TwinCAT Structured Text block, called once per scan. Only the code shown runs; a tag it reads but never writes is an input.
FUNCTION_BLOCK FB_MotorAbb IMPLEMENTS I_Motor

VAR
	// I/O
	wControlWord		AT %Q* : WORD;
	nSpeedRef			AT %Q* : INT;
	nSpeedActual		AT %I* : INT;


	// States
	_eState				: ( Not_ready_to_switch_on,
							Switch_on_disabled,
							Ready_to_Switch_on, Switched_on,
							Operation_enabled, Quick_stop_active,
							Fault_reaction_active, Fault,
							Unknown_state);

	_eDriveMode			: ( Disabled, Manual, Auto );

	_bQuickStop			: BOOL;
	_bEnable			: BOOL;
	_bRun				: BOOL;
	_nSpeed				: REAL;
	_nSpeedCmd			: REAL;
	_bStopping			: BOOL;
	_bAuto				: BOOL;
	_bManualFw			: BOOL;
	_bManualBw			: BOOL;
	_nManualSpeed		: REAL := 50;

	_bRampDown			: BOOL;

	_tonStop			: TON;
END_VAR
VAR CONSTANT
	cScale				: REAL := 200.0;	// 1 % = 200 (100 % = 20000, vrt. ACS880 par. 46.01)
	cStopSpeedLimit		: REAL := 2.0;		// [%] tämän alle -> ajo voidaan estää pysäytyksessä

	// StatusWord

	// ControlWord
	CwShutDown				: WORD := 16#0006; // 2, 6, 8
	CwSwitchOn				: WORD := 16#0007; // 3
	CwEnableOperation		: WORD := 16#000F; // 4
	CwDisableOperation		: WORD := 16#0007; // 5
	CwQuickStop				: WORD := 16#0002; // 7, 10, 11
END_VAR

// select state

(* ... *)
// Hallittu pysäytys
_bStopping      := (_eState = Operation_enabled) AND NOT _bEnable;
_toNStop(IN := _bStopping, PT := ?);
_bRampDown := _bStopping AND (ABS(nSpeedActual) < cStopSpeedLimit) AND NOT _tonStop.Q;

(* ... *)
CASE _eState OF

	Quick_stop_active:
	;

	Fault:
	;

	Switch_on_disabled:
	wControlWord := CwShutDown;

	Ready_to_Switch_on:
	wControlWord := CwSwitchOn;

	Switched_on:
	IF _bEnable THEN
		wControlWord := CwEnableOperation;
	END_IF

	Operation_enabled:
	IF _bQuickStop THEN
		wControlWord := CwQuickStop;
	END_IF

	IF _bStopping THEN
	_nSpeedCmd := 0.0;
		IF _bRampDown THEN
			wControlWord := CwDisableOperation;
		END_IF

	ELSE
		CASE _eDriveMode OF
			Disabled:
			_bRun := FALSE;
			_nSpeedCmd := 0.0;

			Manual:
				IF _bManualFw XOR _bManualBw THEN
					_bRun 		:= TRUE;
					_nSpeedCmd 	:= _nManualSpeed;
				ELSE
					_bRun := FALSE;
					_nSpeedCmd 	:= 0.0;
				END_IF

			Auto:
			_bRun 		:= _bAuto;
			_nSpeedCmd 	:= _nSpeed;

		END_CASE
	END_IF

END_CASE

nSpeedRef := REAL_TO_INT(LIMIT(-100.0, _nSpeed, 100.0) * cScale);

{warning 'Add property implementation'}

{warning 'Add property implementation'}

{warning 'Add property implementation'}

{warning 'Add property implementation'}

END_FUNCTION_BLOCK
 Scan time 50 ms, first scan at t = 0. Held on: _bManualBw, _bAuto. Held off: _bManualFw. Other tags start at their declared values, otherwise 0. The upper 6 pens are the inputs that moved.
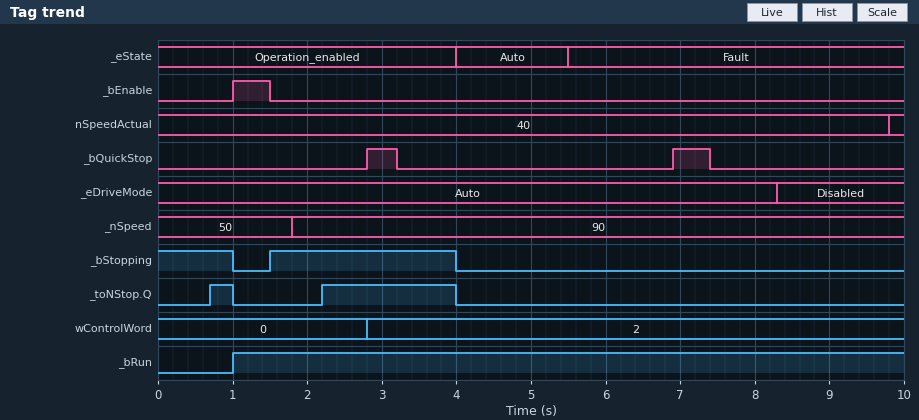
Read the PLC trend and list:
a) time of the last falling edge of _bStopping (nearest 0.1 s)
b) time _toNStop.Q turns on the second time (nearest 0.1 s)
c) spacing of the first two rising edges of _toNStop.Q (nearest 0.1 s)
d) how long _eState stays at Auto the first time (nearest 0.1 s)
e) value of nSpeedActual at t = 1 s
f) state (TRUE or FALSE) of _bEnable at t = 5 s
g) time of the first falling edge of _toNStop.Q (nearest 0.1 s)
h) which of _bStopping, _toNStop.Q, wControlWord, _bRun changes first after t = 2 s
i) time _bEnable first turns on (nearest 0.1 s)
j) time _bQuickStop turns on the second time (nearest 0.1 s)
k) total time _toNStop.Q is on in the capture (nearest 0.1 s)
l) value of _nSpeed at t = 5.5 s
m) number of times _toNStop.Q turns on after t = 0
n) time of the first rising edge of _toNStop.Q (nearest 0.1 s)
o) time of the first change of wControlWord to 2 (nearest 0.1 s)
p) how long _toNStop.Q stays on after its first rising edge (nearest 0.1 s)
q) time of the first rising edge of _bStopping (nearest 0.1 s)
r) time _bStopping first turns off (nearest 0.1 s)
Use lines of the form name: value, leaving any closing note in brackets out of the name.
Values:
time of the last falling edge of _bStopping: 4.0 s
time _toNStop.Q turns on the second time: 2.2 s
spacing of the first two rising edges of _toNStop.Q: 1.5 s
how long _eState stays at Auto the first time: 1.5 s
value of nSpeedActual at t = 1 s: 40
state (TRUE or FALSE) of _bEnable at t = 5 s: FALSE
time of the first falling edge of _toNStop.Q: 1.0 s
which of _bStopping, _toNStop.Q, wControlWord, _bRun changes first after t = 2 s: _toNStop.Q
time _bEnable first turns on: 1.0 s
time _bQuickStop turns on the second time: 6.9 s
total time _toNStop.Q is on in the capture: 2.1 s
value of _nSpeed at t = 5.5 s: 90
number of times _toNStop.Q turns on after t = 0: 2
time of the first rising edge of _toNStop.Q: 0.7 s
time of the first change of wControlWord to 2: 2.8 s
how long _toNStop.Q stays on after its first rising edge: 0.3 s
time of the first rising edge of _bStopping: 1.5 s
time _bStopping first turns off: 1.0 s
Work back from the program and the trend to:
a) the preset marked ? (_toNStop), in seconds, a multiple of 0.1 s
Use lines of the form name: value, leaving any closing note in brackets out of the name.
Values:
the preset marked ? (_toNStop), in seconds, a multiple of 0.1 s: 0.7 s
